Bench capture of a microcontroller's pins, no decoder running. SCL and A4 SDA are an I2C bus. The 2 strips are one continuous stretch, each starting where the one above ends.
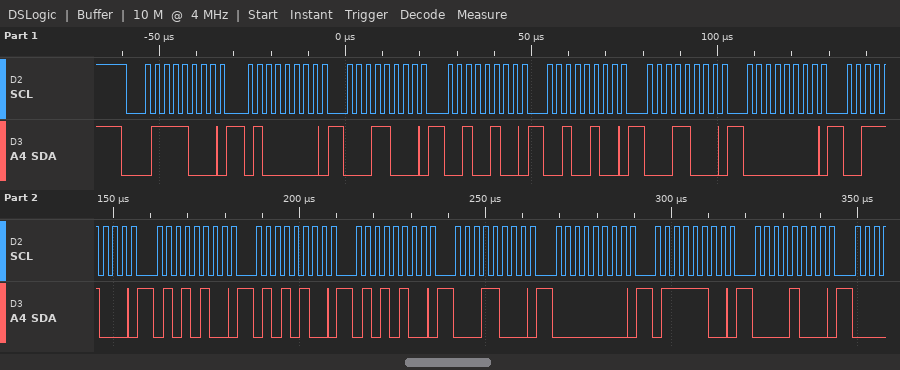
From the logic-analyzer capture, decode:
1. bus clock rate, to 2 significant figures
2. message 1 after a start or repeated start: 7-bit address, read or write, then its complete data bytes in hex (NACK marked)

400 kHz
0x3C write: 40 18 24 24 18 00 38 54 54 54 18 00 7C 08
